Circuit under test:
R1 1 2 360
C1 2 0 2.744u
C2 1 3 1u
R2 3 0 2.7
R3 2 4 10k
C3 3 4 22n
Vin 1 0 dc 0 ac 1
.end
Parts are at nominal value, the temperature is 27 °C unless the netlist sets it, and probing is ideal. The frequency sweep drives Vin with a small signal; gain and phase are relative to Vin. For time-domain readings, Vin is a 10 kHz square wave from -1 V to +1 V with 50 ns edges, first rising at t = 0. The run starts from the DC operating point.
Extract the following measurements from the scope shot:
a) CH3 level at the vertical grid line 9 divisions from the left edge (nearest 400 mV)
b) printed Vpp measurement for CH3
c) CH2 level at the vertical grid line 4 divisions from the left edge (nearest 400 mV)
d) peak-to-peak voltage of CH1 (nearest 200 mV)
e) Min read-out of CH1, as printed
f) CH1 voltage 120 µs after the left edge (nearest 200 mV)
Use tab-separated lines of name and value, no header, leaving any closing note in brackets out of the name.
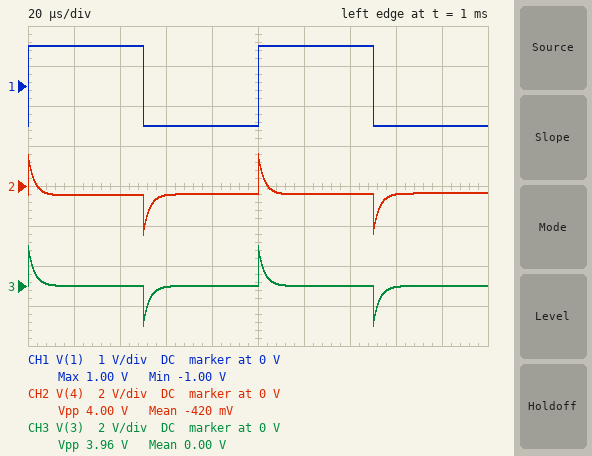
CH3 level at the vertical grid line 9 divisions from the left edge	0 V
printed Vpp measurement for CH3	3.96 V
CH2 level at the vertical grid line 4 divisions from the left edge	-400 mV
peak-to-peak voltage of CH1	2.0 V
Min read-out of CH1, as printed	-1.00 V
CH1 voltage 120 µs after the left edge	1.0 V
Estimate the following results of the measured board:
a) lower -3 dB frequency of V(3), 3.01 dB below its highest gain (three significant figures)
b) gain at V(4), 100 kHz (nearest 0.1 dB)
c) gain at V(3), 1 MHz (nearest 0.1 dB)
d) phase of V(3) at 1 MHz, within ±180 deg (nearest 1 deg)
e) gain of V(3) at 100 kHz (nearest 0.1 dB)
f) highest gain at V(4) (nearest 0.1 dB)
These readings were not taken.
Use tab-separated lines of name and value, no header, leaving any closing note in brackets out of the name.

lower -3 dB frequency of V(3), 3.01 dB below its highest gain	59.0 kHz
gain at V(4), 100 kHz	-1.3 dB
gain at V(3), 1 MHz	0 dB
phase of V(3) at 1 MHz, within ±180 deg	3 deg
gain of V(3) at 100 kHz	-1.3 dB
highest gain at V(4)	0 dB
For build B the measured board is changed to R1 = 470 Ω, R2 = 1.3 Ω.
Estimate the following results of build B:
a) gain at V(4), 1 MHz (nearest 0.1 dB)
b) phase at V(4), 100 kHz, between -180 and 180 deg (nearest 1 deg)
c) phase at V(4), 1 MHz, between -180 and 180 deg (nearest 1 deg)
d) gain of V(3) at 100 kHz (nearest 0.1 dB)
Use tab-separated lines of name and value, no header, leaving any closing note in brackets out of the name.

gain at V(4), 1 MHz	-0.1 dB
phase at V(4), 100 kHz, between -180 and 180 deg	51 deg
phase at V(4), 1 MHz, between -180 and 180 deg	7 deg
gain of V(3) at 100 kHz	-4.0 dB
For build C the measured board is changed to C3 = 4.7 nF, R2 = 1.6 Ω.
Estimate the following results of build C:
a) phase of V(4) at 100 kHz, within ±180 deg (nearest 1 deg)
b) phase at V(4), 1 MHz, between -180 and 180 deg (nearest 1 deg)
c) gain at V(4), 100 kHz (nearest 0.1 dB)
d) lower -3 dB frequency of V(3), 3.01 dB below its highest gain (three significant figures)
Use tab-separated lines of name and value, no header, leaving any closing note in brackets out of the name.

phase of V(4) at 100 kHz, within ±180 deg	47 deg
phase at V(4), 1 MHz, between -180 and 180 deg	6 deg
gain at V(4), 100 kHz	-3.0 dB
lower -3 dB frequency of V(3), 3.01 dB below its highest gain	99.5 kHz
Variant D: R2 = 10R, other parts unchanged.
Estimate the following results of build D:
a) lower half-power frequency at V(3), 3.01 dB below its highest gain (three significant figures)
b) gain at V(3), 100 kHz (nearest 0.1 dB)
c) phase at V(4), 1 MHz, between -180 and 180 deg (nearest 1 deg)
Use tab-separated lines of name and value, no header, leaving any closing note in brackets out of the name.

lower half-power frequency at V(3), 3.01 dB below its highest gain	15.9 kHz
gain at V(3), 100 kHz	-0.1 dB
phase at V(4), 1 MHz, between -180 and 180 deg	1 deg
